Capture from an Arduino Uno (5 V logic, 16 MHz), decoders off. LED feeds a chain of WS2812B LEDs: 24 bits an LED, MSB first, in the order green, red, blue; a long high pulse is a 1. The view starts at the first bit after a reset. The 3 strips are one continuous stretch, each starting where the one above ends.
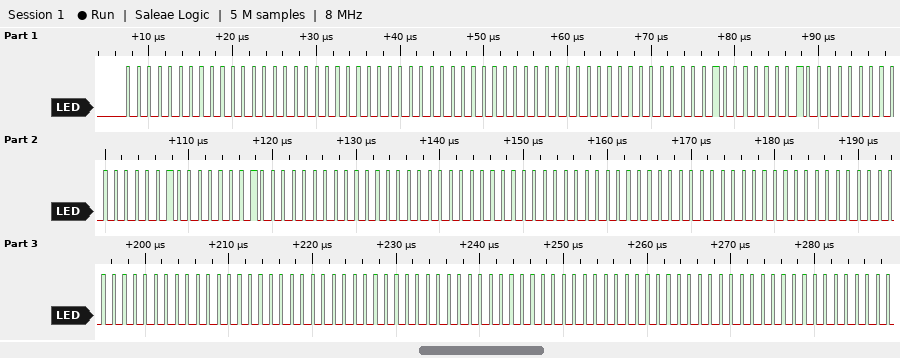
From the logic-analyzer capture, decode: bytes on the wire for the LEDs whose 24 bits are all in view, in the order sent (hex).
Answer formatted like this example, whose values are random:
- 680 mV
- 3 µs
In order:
- 00 00 00 00 00 00 00 80 80 00 80 80 00 00 00 00 00 00 00 00 00 00 00 00 00 00 00
